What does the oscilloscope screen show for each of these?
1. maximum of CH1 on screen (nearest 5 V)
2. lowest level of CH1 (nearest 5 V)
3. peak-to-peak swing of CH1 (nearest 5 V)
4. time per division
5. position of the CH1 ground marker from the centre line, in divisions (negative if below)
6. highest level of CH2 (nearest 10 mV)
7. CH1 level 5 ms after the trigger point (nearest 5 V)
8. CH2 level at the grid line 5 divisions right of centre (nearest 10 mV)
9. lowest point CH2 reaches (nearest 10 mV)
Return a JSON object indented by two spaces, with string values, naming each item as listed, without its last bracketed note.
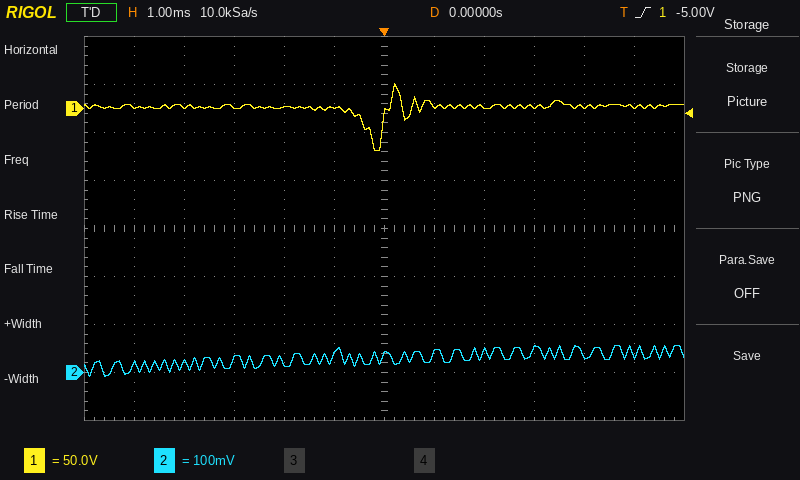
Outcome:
{
  "maximum of CH1 on screen": "25 V",
  "lowest level of CH1": "-45 V",
  "peak-to-peak swing of CH1": "70 V",
  "time per division": "1 ms",
  "position of the CH1 ground marker from the centre line, in divisions": "+2.5 div",
  "highest level of CH2": "60 mV",
  "CH1 level 5 ms after the trigger point": "0 V",
  "CH2 level at the grid line 5 divisions right of centre": "40 mV",
  "lowest point CH2 reaches": "-10 mV"
}
